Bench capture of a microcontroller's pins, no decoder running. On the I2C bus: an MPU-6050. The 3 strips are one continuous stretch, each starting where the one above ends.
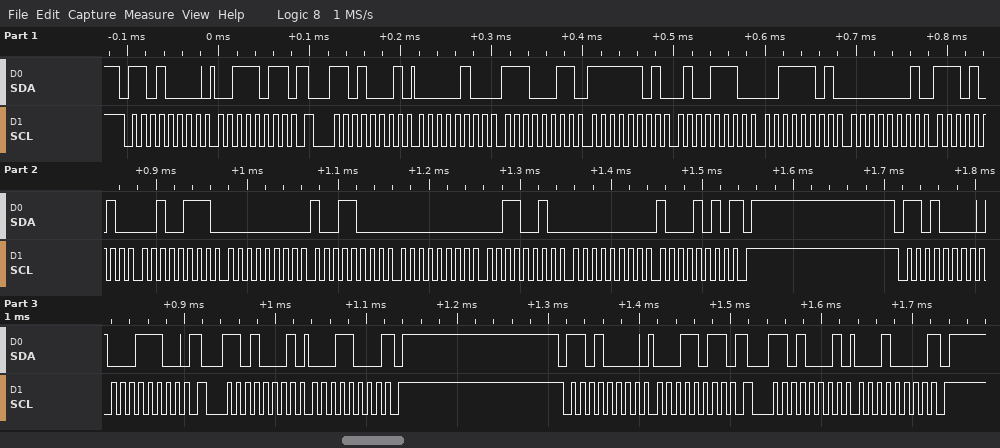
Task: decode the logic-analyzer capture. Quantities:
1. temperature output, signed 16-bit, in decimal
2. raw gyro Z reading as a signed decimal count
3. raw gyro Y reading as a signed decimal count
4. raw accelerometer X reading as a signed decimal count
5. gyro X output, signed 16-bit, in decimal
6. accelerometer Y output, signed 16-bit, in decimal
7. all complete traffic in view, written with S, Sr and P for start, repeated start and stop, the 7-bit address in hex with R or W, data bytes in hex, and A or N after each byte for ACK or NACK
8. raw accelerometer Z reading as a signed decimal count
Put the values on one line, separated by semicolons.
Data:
-5593; 138; 50; 1251; 152; -690; S 68W A 3B A Sr 68R A 04 A E3 A FD A 4E A 3D A 01 A EA A 27 A 00 A 98 A 00 A 32 A 00 A 8A N P S 68W A 1C A Sr 68R A 18 N P S 68W A 1B A Sr 68R A 10 N P; 15617
